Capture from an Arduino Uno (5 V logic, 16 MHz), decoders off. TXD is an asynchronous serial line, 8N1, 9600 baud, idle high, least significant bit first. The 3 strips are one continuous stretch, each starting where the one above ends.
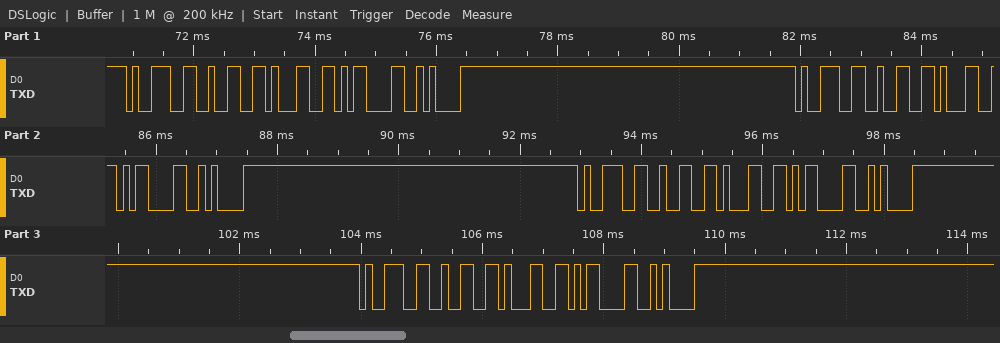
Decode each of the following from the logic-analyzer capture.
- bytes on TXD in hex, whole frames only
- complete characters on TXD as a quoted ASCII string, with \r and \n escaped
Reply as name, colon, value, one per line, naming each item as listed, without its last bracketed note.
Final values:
bytes on TXD in hex, whole frames only: 39 32 31 0D 0A 39 32 31 0D 0A 39 32 31 0D 0A 39 32 31 0D 0A
complete characters on TXD as a quoted ASCII string, with \r and \n escaped: "921\r\n921\r\n921\r\n921\r\n"
